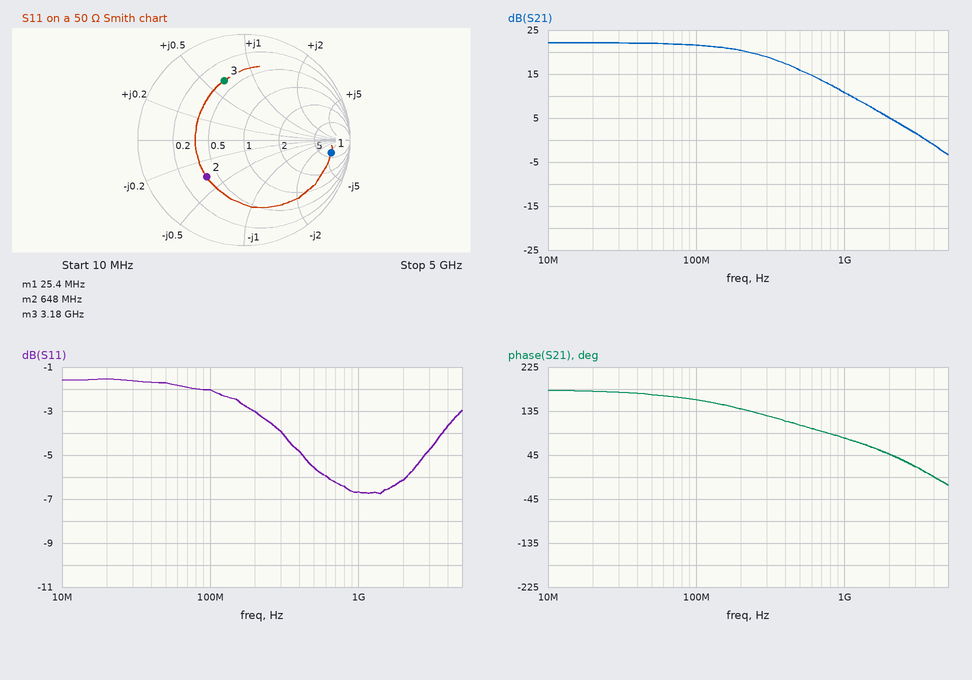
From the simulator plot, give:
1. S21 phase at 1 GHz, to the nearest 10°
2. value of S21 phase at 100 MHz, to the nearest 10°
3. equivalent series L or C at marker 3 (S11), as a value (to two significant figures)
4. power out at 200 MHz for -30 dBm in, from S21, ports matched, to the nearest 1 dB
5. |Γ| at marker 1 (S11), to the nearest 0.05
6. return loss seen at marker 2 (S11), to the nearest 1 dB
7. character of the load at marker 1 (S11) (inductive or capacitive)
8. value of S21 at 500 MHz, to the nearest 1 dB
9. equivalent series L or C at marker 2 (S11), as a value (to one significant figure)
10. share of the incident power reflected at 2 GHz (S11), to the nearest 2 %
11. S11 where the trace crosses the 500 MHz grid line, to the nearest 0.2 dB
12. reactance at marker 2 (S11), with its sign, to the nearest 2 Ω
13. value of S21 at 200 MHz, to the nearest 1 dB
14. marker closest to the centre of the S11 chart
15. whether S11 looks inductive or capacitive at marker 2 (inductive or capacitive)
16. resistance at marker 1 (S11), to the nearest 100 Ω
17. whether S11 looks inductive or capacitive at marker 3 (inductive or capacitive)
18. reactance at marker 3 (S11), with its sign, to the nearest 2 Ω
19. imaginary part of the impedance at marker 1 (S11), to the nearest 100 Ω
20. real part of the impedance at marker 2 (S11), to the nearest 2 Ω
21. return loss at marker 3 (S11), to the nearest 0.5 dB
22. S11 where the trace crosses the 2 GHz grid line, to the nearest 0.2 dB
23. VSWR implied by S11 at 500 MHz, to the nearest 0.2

80°
160°
1.6 nH
-10 dBm
0.85
6 dB
capacitive
16 dB
10 pF
24 %
-5.6 dB
-18 Ω
20 dB
marker 2
capacitive
300 Ω
inductive
+32 Ω
-300 Ω
20 Ω
4.5 dB
-6.2 dB
3.2
